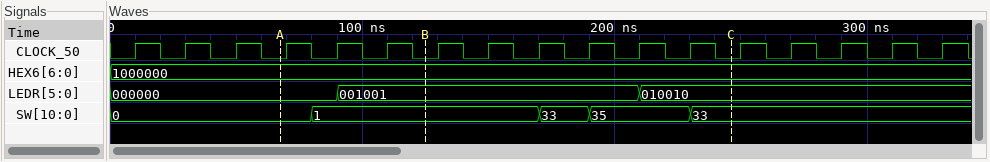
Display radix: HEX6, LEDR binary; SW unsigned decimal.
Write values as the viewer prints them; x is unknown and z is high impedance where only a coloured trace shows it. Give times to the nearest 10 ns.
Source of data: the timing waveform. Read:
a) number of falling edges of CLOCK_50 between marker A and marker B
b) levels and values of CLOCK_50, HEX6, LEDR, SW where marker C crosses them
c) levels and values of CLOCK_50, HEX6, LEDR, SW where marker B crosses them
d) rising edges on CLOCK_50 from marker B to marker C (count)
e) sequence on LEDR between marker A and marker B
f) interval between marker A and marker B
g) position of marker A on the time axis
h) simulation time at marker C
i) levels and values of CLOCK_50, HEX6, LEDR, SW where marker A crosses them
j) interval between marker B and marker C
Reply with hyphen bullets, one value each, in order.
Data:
- 3
- CLOCK_50=0, HEX6=1000000, LEDR=010010, SW=33
- CLOCK_50=0, HEX6=1000000, LEDR=001001, SW=1
- 6
- 000000, 001001
- 60 ns
- 70 ns
- 250 ns
- CLOCK_50=0, HEX6=1000000, LEDR=000000, SW=0
- 120 ns
